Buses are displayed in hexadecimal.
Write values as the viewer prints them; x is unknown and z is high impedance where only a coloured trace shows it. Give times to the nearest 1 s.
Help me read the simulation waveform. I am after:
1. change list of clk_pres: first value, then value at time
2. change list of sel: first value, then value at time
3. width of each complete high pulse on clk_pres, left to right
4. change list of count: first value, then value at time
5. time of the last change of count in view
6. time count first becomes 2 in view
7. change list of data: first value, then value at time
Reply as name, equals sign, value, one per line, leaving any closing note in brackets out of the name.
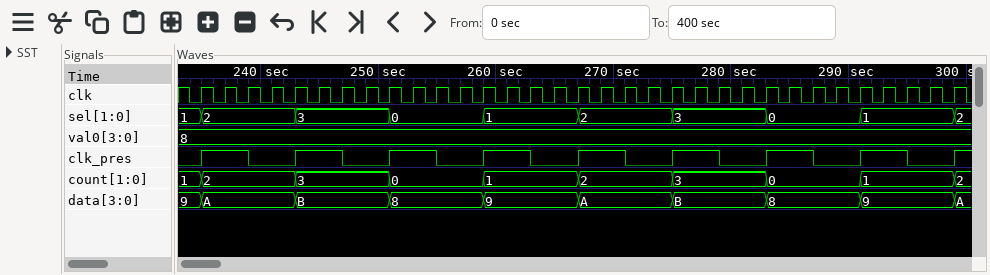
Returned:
change list of clk_pres: first value, then value at time = 0, 1 at 235 s, 0 at 239 s, 1 at 243 s, 0 at 247 s, 1 at 251 s, 0 at 255 s, 1 at 259 s, 0 at 263 s, 1 at 267 s, 0 at 271 s, 1 at 275 s, 0 at 279 s, 1 at 283 s, 0 at 287 s, 1 at 291 s, 0 at 295 s, 1 at 299 s
change list of sel: first value, then value at time = 1, 2 at 235 s, 3 at 243 s, 0 at 251 s, 1 at 259 s, 2 at 267 s, 3 at 275 s, 0 at 283 s, 1 at 291 s, 2 at 299 s
width of each complete high pulse on clk_pres, left to right = 4 s, 4 s, 4 s, 4 s, 4 s, 4 s, 4 s, 4 s
change list of count: first value, then value at time = 1, 2 at 235 s, 3 at 243 s, 0 at 251 s, 1 at 259 s, 2 at 267 s, 3 at 275 s, 0 at 283 s, 1 at 291 s, 2 at 299 s
time of the last change of count in view = 299 s
time count first becomes 2 in view = 235 s
change list of data: first value, then value at time = 9, A at 235 s, B at 243 s, 8 at 251 s, 9 at 259 s, A at 267 s, B at 275 s, 8 at 283 s, 9 at 291 s, A at 299 s
